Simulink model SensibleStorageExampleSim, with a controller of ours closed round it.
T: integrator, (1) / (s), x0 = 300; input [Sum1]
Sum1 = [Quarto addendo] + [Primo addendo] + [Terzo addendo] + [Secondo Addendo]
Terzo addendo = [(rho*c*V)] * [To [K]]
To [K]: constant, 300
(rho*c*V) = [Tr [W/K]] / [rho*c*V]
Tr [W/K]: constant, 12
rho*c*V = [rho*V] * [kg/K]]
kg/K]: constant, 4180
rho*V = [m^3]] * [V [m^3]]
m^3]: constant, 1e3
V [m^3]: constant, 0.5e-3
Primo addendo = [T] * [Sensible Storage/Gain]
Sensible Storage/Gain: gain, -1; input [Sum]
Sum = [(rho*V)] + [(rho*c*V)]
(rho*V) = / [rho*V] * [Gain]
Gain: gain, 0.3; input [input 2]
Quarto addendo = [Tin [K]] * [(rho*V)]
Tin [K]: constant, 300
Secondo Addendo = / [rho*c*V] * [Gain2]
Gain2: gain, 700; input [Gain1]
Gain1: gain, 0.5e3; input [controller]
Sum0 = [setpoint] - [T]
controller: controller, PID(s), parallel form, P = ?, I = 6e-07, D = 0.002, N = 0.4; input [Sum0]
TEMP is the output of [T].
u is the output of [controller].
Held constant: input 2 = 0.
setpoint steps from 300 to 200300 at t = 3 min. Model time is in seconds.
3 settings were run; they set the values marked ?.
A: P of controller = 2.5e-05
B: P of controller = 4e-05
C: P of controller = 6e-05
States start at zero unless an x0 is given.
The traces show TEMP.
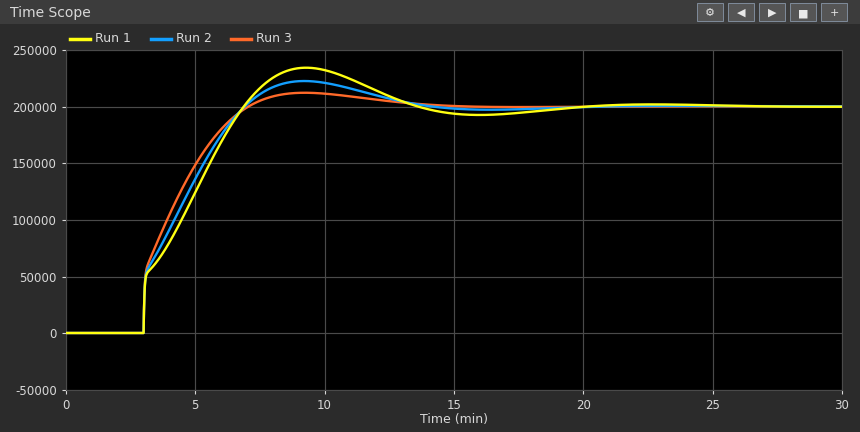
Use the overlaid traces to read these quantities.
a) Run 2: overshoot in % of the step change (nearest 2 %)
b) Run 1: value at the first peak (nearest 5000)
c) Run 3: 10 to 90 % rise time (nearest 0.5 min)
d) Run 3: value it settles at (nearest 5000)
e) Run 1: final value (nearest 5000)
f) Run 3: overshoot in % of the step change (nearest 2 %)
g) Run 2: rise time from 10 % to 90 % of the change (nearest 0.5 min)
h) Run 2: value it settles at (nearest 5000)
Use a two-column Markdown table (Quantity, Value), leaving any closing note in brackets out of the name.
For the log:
| Quantity | Value |
|---|---|
| Run 2: overshoot in % of the step change | 12 % |
| Run 1: value at the first peak | 235000 |
| Run 3: 10 to 90 % rise time | 3.0 min |
| Run 3: value it settles at | 200000 |
| Run 1: final value | 200000 |
| Run 3: overshoot in % of the step change | 6 % |
| Run 2: rise time from 10 % to 90 % of the change | 3.0 min |
| Run 2: value it settles at | 200000 |
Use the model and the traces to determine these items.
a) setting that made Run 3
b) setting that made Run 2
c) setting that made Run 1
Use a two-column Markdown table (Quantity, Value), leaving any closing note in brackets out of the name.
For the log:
| Quantity | Value |
|---|---|
| setting that made Run 3 | C |
| setting that made Run 2 | B |
| setting that made Run 1 | A |
